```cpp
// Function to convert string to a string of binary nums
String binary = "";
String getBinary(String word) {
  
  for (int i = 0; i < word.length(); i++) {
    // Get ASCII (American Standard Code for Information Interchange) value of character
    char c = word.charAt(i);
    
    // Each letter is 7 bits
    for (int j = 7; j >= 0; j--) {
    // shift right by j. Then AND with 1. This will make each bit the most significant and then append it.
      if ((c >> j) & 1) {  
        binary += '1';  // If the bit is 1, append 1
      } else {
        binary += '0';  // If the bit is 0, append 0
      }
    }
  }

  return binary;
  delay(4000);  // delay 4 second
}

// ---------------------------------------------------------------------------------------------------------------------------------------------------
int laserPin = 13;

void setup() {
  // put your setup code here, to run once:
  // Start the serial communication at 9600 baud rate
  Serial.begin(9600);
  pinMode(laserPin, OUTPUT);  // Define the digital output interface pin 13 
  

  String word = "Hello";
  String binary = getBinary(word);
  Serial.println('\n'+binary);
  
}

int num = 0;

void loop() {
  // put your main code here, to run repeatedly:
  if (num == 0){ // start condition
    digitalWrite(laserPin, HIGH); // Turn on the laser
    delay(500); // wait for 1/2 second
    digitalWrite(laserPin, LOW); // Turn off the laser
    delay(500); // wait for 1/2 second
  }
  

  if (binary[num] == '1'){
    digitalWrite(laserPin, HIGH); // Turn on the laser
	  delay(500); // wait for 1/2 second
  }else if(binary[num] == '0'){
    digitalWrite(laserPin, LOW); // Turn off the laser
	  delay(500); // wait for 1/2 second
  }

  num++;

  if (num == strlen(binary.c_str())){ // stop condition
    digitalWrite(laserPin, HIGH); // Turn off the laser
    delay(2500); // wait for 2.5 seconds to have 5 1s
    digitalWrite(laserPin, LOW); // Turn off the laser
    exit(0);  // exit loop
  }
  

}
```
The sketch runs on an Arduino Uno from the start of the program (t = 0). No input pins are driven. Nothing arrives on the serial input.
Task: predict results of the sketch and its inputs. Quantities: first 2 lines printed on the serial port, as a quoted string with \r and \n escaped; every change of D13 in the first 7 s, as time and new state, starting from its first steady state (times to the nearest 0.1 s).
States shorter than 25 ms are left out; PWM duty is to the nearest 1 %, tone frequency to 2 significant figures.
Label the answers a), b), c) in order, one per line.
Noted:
a) "\n0100100001100101011011000110110001101111\r\n"
b) 0 s high; 0.5 s low; 1.5 s high; 2 s low; 3 s high; 3.5 s low; 5.5 s high; 6.5 s low
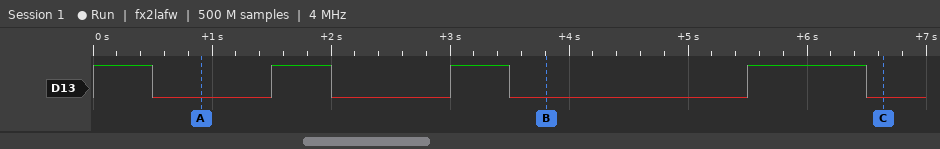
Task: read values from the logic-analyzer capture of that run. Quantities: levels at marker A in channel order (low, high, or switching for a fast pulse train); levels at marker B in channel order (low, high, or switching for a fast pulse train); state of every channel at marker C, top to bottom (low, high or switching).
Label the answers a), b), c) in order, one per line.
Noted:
a) D13 low
b) D13 low
c) D13 low
